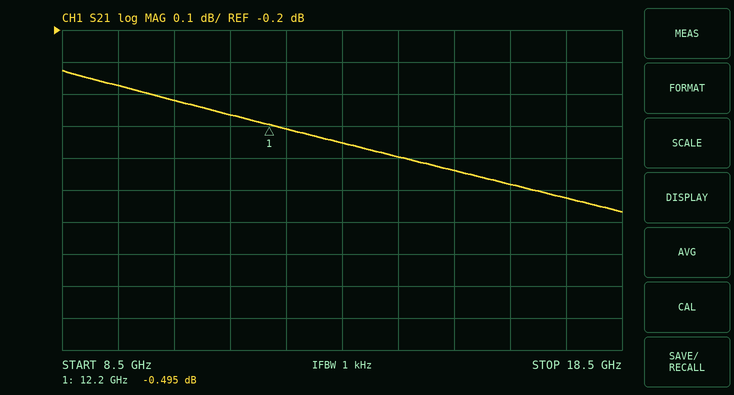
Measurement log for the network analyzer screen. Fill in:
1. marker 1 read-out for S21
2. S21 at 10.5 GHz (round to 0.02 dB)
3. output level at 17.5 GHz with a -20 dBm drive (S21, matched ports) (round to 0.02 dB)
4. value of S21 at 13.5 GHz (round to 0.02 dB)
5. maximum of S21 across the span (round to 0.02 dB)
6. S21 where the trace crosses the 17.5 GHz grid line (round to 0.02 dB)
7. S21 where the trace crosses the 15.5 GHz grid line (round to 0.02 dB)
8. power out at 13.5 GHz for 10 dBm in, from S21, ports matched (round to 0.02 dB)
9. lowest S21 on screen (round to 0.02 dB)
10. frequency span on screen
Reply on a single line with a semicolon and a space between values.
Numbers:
-0.495 dB; -0.42 dB; -20.72 dBm; -0.56 dB; -0.32 dB; -0.72 dB; -0.64 dB; 9.44 dBm; -0.76 dB; 10 GHz
